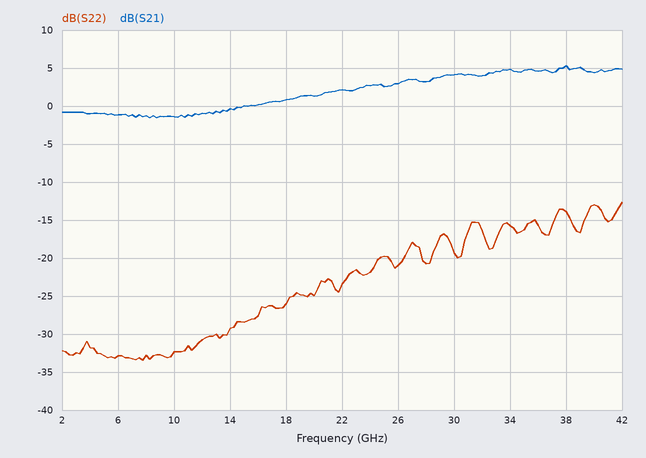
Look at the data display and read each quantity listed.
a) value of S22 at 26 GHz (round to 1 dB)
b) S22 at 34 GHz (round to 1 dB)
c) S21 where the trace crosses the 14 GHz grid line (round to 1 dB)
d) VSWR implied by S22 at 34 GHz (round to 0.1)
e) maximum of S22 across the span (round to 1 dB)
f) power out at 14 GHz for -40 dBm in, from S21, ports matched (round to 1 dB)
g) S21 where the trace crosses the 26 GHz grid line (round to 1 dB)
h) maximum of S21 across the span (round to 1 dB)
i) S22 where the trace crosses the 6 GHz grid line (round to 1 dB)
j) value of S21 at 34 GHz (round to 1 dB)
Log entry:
-21 dB
-16 dB
0 dB
1.4
-13 dB
-40 dBm
3 dB
5 dB
-33 dB
5 dB
